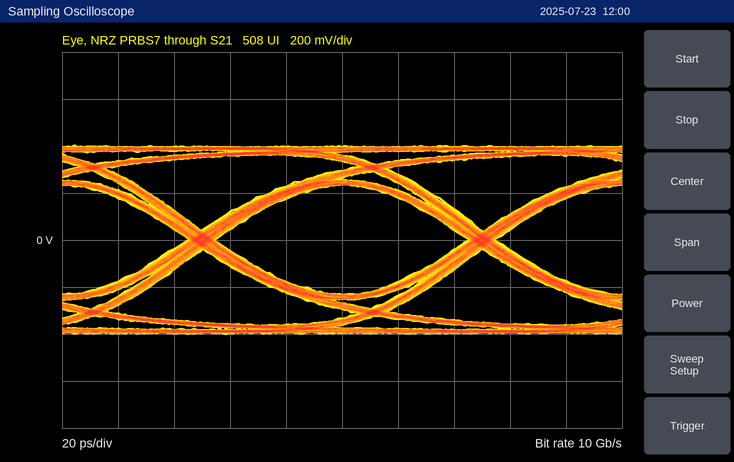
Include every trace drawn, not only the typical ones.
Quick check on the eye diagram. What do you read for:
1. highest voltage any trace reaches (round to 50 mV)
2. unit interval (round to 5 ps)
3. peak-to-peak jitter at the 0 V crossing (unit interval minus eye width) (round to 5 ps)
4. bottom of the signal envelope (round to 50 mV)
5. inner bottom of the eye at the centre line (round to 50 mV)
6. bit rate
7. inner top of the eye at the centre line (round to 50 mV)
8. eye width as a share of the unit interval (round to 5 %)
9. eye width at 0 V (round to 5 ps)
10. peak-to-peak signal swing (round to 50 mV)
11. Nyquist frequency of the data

400 mV
100 ps
10 ps
-400 mV
-250 mV
10 Gb/s
250 mV
90 %
90 ps
800 mV
5 GHz
